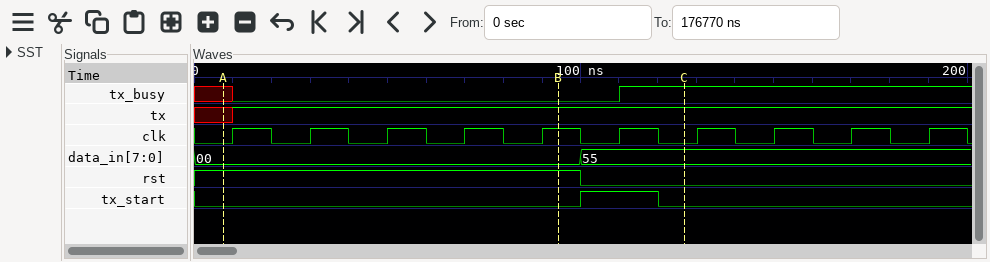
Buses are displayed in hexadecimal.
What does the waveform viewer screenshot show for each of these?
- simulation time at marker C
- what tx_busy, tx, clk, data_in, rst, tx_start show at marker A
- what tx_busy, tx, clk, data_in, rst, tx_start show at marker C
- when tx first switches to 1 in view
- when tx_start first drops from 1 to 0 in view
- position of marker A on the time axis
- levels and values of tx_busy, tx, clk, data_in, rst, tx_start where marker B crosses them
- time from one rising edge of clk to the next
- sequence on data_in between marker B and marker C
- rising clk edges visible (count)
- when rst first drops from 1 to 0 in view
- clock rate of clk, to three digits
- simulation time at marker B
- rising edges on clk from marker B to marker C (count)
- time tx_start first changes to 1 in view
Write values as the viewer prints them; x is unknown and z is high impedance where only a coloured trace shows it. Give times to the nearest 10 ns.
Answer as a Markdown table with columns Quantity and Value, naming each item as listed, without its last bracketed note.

| Quantity | Value |
|---|---|
| simulation time at marker C | 130 ns |
| what tx_busy, tx, clk, data_in, rst, tx_start show at marker A | tx_busy=x, tx=x, clk=0, data_in=00, rst=1, tx_start=0 |
| what tx_busy, tx, clk, data_in, rst, tx_start show at marker C | tx_busy=1, tx=1, clk=0, data_in=55, rst=0, tx_start=0 |
| when tx first switches to 1 in view | 10 ns |
| when tx_start first drops from 1 to 0 in view | 120 ns |
| position of marker A on the time axis | 10 ns |
| levels and values of tx_busy, tx, clk, data_in, rst, tx_start where marker B crosses them | tx_busy=0, tx=1, clk=1, data_in=00, rst=1, tx_start=0 |
| time from one rising edge of clk to the next | 20 ns |
| sequence on data_in between marker B and marker C | 00, 55 |
| rising clk edges visible | 10 |
| when rst first drops from 1 to 0 in view | 100 ns |
| clock rate of clk, to three digits | 50.0 MHz |
| simulation time at marker B | 90 ns |
| rising edges on clk from marker B to marker C | 1 |
| time tx_start first changes to 1 in view | 100 ns |
